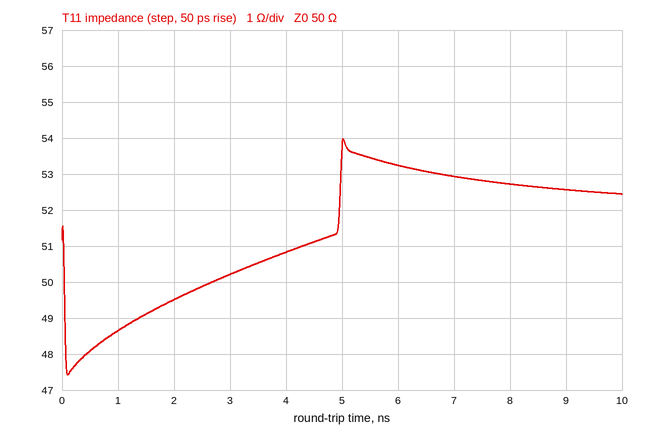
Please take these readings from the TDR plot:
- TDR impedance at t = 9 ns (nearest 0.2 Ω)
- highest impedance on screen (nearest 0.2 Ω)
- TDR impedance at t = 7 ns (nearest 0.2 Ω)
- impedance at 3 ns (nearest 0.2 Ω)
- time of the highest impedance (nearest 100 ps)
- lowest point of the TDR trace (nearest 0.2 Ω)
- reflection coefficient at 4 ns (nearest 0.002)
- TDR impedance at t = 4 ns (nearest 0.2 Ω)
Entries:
52.6 Ω
54.0 Ω
53.0 Ω
50.2 Ω
5.0 ns
47.4 Ω
+0.008
50.8 Ω
